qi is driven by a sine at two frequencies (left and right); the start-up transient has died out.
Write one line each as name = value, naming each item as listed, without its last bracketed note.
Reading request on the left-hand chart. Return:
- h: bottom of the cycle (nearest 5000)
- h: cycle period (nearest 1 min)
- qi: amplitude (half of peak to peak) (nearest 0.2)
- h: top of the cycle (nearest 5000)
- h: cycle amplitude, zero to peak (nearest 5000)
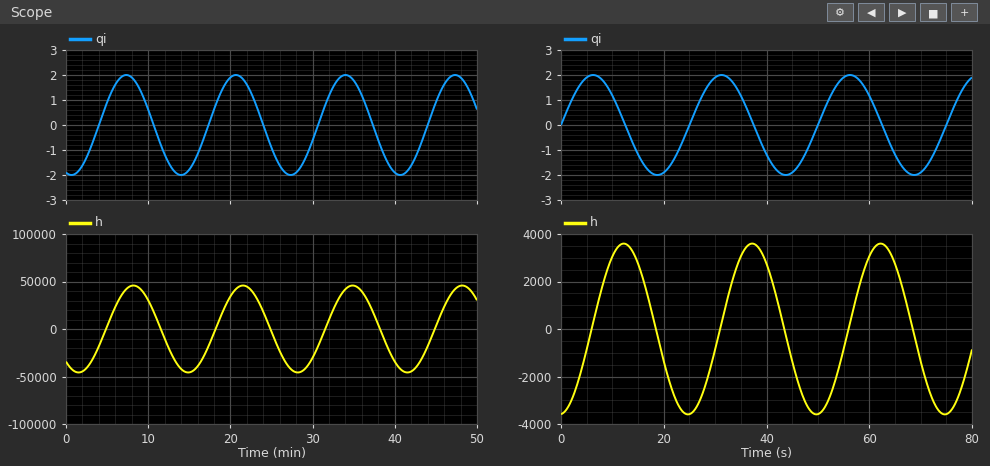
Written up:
h: bottom of the cycle = -45000
h: cycle period = 13 min
qi: amplitude (half of peak to peak) = 2.0
h: top of the cycle = 45000
h: cycle amplitude, zero to peak = 45000
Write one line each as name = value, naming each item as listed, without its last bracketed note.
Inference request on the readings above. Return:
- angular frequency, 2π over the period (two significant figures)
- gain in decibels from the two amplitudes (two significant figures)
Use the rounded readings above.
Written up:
angular frequency, 2π over the period = 0.48 rad/min
gain in decibels from the two amplitudes = 87 dB
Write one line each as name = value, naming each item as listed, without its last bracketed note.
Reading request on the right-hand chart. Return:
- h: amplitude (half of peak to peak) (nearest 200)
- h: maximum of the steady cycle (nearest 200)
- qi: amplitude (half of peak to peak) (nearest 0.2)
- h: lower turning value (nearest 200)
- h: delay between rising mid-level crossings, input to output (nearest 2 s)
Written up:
h: amplitude (half of peak to peak) = 3600
h: maximum of the steady cycle = 3600
qi: amplitude (half of peak to peak) = 2.0
h: lower turning value = -3600
h: delay between rising mid-level crossings, input to output = 6 s
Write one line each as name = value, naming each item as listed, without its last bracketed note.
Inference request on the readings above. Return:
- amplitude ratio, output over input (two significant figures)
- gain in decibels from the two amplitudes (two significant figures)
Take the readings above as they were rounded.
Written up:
amplitude ratio, output over input = 1800
gain in decibels from the two amplitudes = 65 dB
